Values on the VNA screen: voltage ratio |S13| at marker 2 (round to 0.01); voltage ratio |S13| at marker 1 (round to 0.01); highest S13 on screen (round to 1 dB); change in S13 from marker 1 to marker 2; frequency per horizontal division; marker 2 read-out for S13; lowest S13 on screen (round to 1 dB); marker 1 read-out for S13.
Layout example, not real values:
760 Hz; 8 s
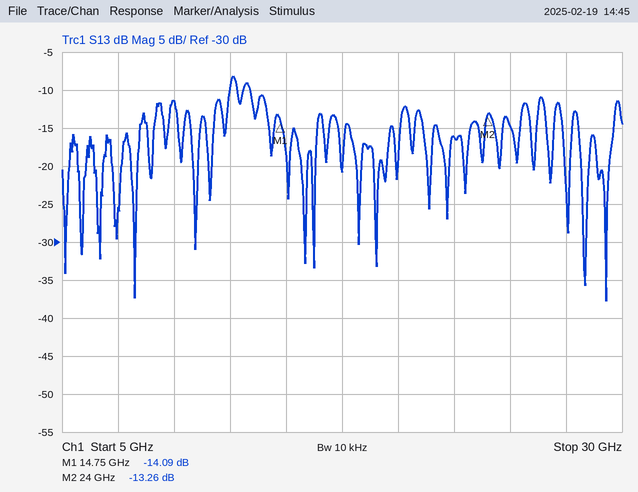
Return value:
0.22; 0.20; -8 dB; 0.83 dB; 2.5 GHz; -13.26 dB; -38 dB; -14.09 dB
